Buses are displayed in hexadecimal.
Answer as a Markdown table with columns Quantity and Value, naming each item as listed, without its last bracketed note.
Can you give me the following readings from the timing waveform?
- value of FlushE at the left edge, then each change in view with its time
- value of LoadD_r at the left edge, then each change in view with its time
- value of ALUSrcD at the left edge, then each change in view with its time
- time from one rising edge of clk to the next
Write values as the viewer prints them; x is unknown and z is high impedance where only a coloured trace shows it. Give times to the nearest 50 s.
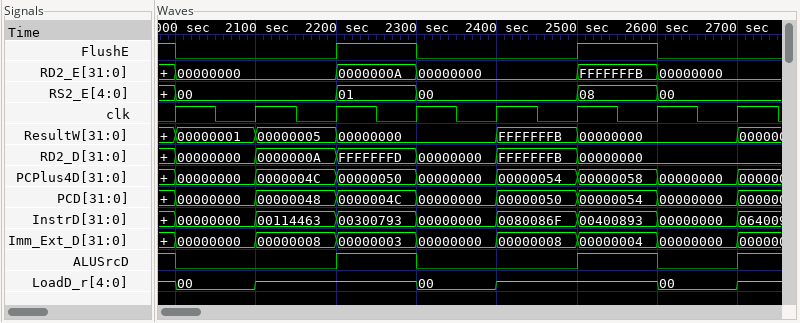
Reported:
| Quantity | Value |
|---|---|
| value of FlushE at the left edge, then each change in view with its time | 1, 0 at 2000 s, 1 at 2200 s, 0 at 2300 s, 1 at 2500 s, 0 at 2600 s |
| value of LoadD_r at the left edge, then each change in view with its time | z, 00 at 2000 s, z at 2100 s, 00 at 2300 s, z at 2400 s, 00 at 2600 s, z at 2700 s |
| value of ALUSrcD at the left edge, then each change in view with its time | 1, 0 at 2000 s, 1 at 2200 s, 0 at 2300 s, 1 at 2500 s, 0 at 2600 s, 1 at 2700 s |
| time from one rising edge of clk to the next | 100 s |
